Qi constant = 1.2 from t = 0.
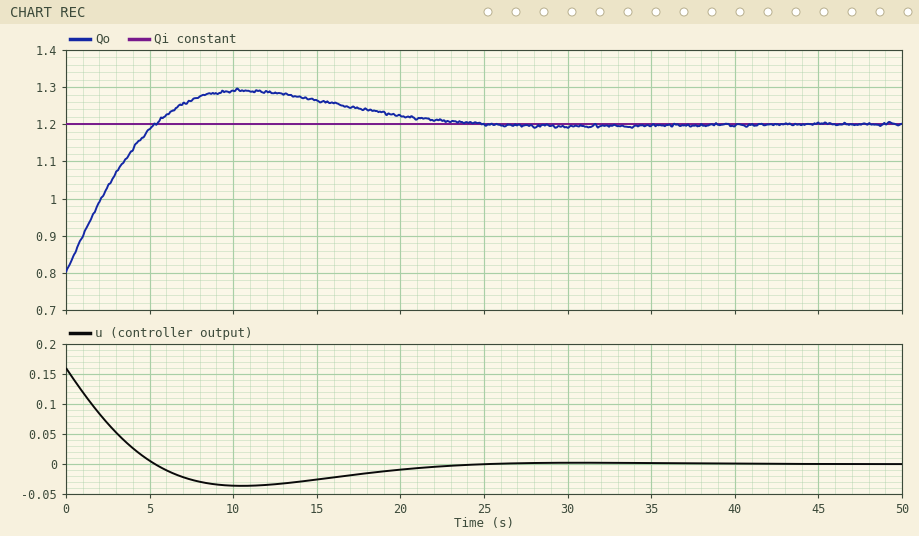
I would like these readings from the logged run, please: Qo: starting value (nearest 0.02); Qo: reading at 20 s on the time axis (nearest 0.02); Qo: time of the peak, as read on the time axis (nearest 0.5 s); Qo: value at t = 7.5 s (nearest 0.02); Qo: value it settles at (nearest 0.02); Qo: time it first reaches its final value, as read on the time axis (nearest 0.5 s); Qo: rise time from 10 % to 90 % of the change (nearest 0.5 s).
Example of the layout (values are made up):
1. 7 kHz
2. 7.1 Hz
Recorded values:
1. 0.80
2. 1.22
3. 10.5 s
4. 1.26
5. 1.20
6. 5.5 s
7. 4.0 s
